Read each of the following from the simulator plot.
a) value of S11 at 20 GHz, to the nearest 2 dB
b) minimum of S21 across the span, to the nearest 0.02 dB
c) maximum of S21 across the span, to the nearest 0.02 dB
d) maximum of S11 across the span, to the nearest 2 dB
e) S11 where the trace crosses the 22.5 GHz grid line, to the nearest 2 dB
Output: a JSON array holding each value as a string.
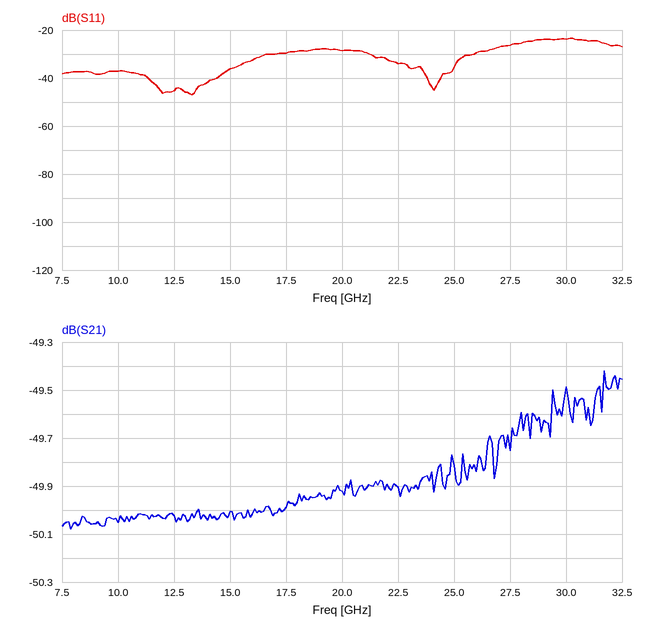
["-28 dB", "-50.08 dB", "-49.42 dB", "-24 dB", "-34 dB"]
